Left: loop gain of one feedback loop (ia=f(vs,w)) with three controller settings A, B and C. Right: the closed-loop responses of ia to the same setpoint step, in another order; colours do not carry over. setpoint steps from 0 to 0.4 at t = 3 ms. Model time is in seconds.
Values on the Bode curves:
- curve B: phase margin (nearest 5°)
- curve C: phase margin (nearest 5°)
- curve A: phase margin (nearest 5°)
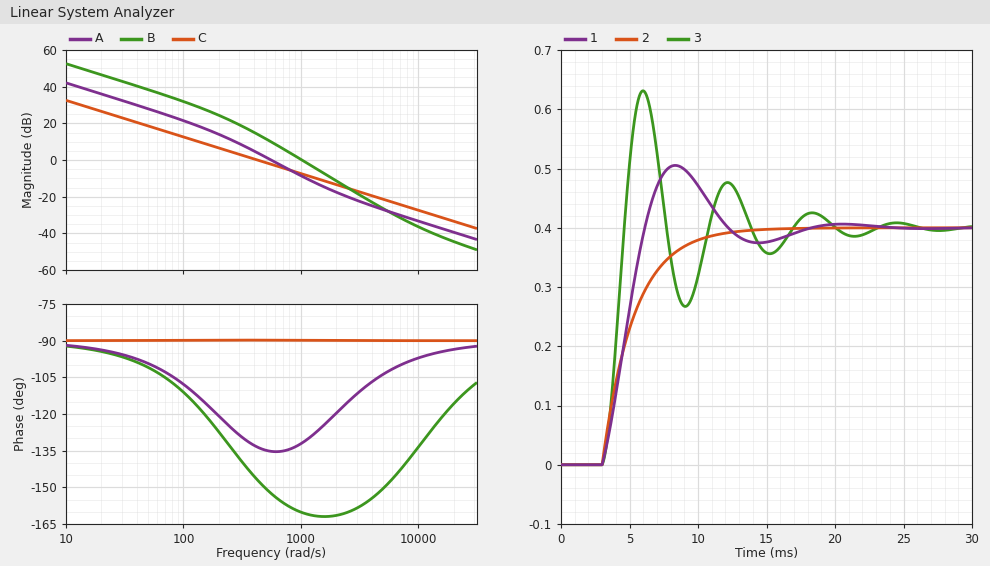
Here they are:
20°
90°
45°
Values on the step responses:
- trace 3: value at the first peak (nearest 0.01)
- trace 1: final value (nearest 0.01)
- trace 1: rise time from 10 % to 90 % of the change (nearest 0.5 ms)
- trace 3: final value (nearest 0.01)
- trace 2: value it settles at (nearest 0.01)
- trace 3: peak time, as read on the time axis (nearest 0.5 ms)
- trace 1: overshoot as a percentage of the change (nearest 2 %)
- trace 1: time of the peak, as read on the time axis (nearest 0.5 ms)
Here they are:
0.63
0.40
2.5 ms
0.40
0.40
6.0 ms
26 %
8.5 ms
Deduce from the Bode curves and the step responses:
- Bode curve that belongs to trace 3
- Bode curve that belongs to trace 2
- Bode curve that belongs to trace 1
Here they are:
B
C
A
